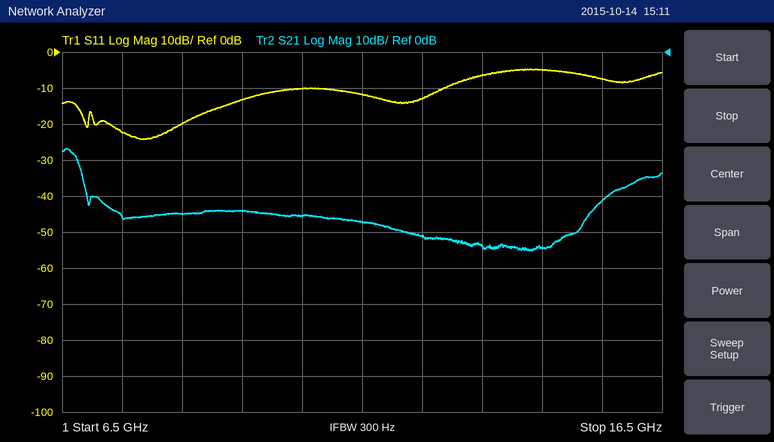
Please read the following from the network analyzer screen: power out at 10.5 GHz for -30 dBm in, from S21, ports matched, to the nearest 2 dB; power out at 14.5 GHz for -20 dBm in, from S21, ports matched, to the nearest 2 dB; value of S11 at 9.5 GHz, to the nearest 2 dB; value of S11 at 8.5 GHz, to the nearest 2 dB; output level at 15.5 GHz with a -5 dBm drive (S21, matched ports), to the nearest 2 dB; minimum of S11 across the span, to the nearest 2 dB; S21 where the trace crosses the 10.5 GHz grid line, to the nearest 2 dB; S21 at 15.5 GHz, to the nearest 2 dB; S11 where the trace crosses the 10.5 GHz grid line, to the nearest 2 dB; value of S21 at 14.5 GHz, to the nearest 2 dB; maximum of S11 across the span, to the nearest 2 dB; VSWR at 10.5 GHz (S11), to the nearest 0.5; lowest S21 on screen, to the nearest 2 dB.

-76 dBm
-74 dBm
-14 dB
-20 dB
-46 dBm
-24 dB
-46 dB
-42 dB
-10 dB
-54 dB
-4 dB
2.0
-56 dB
